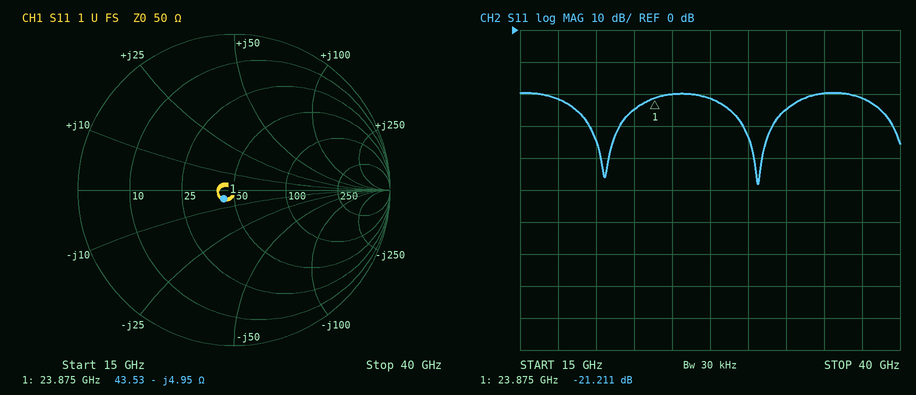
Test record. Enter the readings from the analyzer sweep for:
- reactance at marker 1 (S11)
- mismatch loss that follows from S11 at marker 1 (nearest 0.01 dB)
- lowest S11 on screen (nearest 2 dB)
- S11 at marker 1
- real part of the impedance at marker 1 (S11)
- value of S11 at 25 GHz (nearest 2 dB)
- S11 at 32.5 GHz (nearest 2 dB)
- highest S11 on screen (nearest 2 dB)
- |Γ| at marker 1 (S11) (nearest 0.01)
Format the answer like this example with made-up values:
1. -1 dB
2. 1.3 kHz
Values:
1. -4.95 Ω
2. 0.03 dB
3. -48 dB
4. -21.211 dB
5. 43.53 Ω
6. -20 dB
7. -24 dB
8. -20 dB
9. 0.09
